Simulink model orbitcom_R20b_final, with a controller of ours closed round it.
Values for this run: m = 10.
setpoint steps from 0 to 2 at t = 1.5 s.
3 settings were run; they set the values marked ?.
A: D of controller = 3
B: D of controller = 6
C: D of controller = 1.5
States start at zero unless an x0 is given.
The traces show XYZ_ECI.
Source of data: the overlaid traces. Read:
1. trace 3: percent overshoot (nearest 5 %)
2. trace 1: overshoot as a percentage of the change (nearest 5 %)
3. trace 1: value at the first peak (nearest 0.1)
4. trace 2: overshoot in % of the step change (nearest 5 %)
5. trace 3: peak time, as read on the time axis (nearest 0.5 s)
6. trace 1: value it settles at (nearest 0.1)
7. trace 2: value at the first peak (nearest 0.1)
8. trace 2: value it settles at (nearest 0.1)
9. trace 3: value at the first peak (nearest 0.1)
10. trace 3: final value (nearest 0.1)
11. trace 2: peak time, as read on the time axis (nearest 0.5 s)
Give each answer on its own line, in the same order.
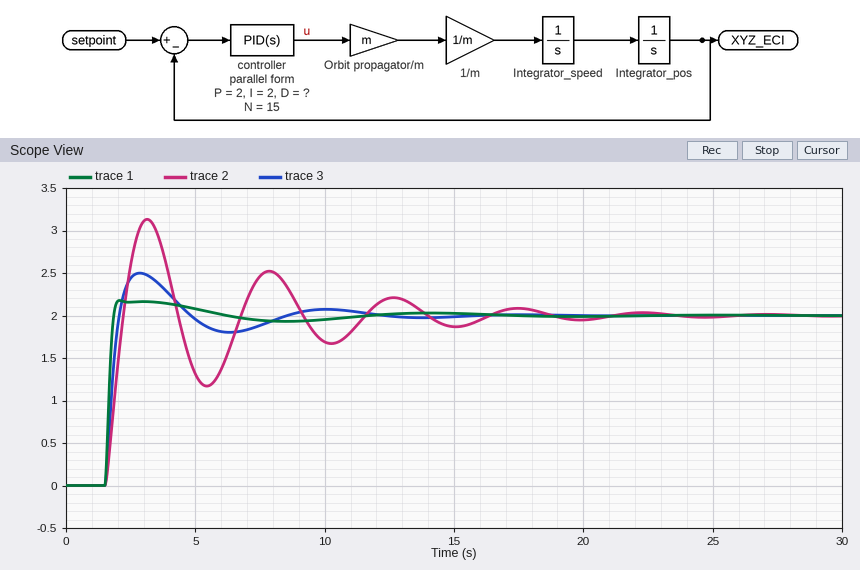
25 %
10 %
2.2
55 %
3.0 s
2.0
3.1
2.0
2.5
2.0
3.0 s
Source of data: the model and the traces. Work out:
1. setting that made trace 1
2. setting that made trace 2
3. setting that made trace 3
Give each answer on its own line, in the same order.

B
C
A
